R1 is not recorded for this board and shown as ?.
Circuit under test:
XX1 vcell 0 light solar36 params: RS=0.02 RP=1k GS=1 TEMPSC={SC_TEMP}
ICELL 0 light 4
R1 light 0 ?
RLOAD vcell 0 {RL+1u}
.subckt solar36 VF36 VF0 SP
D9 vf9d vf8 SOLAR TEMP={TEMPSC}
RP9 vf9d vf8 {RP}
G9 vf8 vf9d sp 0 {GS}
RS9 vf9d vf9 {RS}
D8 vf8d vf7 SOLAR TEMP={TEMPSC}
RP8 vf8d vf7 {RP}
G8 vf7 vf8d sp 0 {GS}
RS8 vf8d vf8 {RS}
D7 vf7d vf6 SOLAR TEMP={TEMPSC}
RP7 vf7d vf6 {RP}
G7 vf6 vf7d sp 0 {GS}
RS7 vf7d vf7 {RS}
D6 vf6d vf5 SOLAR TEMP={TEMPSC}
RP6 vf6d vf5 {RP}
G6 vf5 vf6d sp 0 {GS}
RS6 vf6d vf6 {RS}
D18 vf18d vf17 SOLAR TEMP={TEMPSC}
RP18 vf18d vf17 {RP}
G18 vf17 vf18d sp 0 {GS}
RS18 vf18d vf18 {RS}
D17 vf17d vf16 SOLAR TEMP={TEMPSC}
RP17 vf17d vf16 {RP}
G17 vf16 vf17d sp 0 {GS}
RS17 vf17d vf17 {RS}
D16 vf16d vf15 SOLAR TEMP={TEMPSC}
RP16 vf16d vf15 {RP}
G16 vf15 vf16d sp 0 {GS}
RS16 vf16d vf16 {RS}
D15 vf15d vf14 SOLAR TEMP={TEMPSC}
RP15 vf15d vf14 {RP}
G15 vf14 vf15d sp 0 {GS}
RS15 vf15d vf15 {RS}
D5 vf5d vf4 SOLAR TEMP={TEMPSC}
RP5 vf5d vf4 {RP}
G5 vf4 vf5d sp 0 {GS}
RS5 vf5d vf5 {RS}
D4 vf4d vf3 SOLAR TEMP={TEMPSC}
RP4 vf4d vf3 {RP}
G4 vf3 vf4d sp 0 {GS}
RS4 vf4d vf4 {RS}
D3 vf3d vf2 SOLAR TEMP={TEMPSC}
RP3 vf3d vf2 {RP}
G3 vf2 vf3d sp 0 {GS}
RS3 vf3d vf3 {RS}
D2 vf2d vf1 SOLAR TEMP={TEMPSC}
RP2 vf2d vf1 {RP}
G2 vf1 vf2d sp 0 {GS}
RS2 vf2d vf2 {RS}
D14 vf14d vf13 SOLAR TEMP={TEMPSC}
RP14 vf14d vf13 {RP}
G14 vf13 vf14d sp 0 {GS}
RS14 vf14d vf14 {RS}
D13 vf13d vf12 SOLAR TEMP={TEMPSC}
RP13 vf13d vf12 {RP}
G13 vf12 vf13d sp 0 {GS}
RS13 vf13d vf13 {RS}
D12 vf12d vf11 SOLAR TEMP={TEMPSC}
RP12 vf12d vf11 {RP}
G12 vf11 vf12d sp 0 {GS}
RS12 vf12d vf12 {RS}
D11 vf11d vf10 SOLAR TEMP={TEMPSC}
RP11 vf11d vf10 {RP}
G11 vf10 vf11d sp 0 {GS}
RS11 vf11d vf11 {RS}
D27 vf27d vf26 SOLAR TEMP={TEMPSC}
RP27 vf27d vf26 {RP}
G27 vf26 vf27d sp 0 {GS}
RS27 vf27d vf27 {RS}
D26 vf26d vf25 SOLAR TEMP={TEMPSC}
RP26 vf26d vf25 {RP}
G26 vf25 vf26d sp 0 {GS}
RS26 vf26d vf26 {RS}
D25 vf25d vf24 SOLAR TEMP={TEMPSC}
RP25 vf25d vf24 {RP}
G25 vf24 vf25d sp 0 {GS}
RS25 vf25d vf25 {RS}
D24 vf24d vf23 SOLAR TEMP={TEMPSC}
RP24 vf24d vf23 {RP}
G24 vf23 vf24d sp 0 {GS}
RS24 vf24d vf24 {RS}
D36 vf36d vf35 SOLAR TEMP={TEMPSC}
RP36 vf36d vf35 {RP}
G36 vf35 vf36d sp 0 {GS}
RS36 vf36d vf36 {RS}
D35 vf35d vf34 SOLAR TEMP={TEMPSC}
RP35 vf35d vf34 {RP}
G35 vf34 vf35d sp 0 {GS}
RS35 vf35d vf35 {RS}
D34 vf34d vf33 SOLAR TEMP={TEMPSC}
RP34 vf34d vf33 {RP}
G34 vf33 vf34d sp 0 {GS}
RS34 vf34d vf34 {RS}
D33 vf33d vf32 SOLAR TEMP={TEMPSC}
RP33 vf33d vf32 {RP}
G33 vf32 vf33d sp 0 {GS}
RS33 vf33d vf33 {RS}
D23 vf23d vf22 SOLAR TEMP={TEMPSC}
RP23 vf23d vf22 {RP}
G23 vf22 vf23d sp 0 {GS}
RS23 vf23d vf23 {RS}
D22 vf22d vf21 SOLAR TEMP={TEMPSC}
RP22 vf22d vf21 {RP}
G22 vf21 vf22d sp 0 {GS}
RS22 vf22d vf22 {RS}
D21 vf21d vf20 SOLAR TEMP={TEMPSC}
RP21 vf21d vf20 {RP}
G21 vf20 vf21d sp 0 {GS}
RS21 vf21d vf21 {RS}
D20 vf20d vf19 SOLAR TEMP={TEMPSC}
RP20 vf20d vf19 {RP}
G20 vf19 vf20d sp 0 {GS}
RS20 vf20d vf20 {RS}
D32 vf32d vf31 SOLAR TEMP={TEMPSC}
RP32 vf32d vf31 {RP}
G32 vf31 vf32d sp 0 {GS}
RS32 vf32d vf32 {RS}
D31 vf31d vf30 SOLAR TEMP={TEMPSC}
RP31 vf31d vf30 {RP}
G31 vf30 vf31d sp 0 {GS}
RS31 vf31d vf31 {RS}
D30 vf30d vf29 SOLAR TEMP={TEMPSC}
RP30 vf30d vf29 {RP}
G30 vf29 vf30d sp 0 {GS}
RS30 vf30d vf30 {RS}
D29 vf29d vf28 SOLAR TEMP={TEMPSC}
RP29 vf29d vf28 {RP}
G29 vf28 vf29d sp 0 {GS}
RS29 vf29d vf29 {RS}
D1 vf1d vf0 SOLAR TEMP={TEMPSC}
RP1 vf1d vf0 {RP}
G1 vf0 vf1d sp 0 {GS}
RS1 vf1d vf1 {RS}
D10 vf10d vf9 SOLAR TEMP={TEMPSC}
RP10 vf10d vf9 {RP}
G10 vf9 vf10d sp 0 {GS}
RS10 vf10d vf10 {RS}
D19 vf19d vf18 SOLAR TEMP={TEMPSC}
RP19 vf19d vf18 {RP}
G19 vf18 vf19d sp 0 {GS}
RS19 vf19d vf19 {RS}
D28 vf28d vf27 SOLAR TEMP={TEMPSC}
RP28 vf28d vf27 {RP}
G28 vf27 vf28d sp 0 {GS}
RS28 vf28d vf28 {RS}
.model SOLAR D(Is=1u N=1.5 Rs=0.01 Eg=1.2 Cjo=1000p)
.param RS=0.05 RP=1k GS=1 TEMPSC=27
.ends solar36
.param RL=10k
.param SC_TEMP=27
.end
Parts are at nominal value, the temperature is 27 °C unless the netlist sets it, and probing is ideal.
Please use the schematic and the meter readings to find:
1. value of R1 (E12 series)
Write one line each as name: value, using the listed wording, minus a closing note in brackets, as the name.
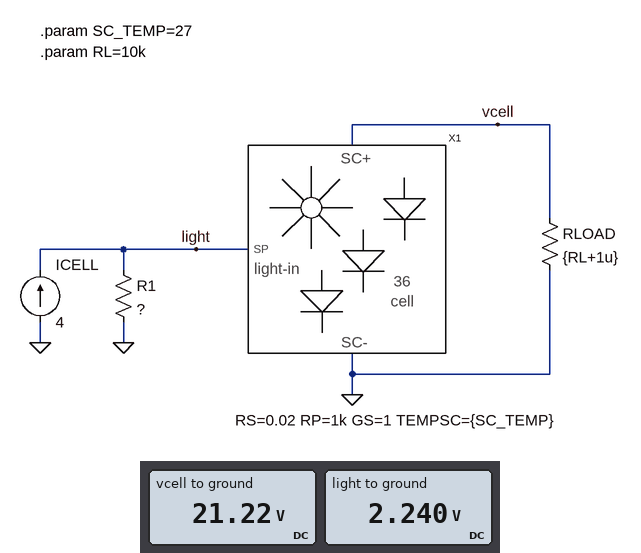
value of R1: 0.56 Ω
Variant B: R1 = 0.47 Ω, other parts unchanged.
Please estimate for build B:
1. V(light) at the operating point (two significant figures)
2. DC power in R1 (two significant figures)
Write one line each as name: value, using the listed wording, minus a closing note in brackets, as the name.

V(light) at the operating point: 1.9 V
DC power in R1: 7.5 W
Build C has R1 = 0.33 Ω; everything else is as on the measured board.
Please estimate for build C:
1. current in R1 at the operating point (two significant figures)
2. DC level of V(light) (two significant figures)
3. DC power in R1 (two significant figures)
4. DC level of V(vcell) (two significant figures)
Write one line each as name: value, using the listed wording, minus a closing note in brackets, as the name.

current in R1 at the operating point: 4.0 A
DC level of V(light): 1.3 V
DC power in R1: 5.3 W
DC level of V(vcell): 20 V
